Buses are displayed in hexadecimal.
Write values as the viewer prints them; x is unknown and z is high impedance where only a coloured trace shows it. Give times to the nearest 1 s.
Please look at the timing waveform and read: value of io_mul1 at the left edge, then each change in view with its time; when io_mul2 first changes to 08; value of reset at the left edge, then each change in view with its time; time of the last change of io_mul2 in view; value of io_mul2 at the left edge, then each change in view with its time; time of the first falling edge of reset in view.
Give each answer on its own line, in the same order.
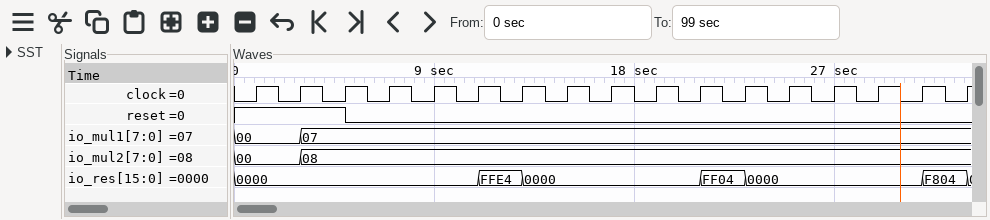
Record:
00, 07 at 3 s
3 s
1, 0 at 5 s
3 s
00, 08 at 3 s
5 s
